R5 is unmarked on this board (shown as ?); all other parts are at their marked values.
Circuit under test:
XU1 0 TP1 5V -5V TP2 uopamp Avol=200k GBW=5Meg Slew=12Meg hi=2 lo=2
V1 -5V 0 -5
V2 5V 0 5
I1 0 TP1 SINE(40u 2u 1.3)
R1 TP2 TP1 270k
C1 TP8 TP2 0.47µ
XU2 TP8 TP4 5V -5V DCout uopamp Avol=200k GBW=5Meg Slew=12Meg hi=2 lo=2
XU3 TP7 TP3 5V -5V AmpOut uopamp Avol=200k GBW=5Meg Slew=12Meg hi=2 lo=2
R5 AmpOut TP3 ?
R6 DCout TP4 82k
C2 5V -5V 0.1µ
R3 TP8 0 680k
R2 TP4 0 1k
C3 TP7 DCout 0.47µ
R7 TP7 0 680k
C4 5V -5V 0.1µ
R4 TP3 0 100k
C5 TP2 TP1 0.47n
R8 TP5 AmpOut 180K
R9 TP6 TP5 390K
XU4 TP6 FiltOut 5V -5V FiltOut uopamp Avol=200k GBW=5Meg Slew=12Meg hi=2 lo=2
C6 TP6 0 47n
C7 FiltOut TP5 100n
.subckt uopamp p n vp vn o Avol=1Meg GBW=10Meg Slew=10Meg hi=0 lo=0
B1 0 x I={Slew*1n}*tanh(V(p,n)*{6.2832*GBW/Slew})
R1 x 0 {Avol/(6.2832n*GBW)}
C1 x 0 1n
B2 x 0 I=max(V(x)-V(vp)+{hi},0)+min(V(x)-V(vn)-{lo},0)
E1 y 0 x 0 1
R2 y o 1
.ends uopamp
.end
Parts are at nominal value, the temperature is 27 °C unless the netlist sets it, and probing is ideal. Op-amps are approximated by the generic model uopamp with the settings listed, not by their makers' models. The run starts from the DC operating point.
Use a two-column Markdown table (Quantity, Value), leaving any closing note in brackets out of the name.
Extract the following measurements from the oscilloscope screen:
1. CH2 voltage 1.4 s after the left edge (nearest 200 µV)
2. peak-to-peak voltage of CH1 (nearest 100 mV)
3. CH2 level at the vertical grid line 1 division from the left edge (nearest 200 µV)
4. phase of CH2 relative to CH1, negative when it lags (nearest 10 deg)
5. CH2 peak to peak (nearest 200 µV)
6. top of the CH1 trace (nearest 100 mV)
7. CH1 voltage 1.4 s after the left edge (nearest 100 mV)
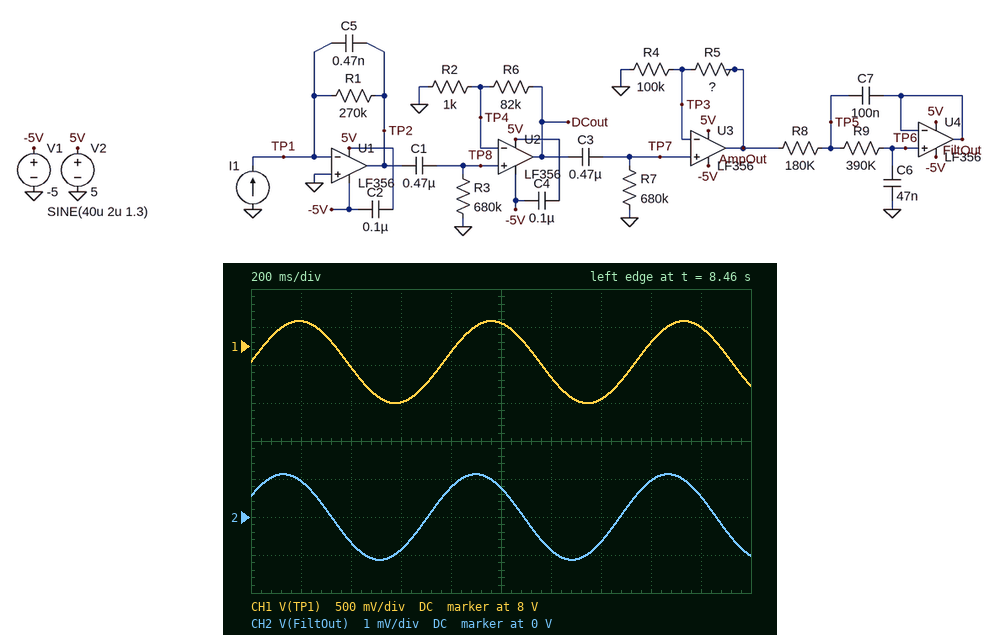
| Quantity | Value |
|---|---|
| CH2 voltage 1.4 s after the left edge | -600 µV |
| peak-to-peak voltage of CH1 | 1.1 V |
| CH2 level at the vertical grid line 1 division from the left edge | 1.0 mV |
| phase of CH2 relative to CH1, negative when it lags | 30 deg |
| CH2 peak to peak | 2.2 mV |
| top of the CH1 trace | 8.3 V |
| CH1 voltage 1.4 s after the left edge | 7.3 V |
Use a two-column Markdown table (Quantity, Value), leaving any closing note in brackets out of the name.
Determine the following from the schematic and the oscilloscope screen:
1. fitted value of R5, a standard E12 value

| Quantity | Value |
|---|---|
| fitted value of R5, a standard E12 value | 680 kΩ |
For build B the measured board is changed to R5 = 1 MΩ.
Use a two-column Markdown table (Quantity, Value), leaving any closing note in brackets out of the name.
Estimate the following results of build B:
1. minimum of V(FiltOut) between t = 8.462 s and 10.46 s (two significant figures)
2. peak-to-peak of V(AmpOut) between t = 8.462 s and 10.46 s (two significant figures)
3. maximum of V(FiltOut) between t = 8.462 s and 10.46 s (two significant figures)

| Quantity | Value |
|---|---|
| minimum of V(FiltOut) between t = 8.462 s and 10.46 s | -1.6 mV |
| peak-to-peak of V(AmpOut) between t = 8.462 s and 10.46 s | 3.2 mV |
| maximum of V(FiltOut) between t = 8.462 s and 10.46 s | 1.6 mV |
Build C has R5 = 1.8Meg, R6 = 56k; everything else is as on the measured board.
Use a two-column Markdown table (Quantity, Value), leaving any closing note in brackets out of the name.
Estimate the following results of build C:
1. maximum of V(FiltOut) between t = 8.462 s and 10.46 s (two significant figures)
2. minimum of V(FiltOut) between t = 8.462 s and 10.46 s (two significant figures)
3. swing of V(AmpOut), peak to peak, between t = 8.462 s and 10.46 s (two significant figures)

| Quantity | Value |
|---|---|
| maximum of V(FiltOut) between t = 8.462 s and 10.46 s | 1.9 mV |
| minimum of V(FiltOut) between t = 8.462 s and 10.46 s | -1.9 mV |
| swing of V(AmpOut), peak to peak, between t = 8.462 s and 10.46 s | 3.8 mV |
